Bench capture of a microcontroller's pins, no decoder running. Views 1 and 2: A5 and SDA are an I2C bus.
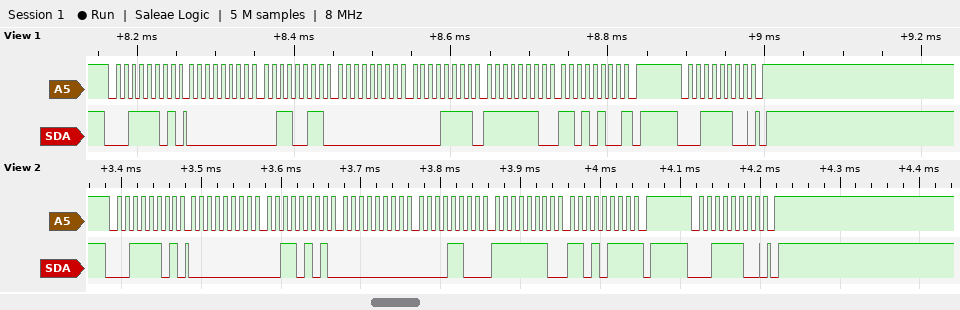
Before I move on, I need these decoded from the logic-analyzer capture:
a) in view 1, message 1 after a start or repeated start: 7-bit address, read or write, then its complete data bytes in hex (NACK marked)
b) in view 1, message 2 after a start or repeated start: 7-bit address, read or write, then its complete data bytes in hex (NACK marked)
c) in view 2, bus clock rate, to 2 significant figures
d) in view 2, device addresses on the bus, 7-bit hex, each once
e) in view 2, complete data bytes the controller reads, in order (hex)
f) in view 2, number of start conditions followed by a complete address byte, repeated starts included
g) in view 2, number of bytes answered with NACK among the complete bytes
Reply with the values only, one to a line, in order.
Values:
0x1E read: 00 33 00 0F FE D4 NACK
0x1E write
100 kHz
0x1E
00 35 00 0C FE D7
2
1
